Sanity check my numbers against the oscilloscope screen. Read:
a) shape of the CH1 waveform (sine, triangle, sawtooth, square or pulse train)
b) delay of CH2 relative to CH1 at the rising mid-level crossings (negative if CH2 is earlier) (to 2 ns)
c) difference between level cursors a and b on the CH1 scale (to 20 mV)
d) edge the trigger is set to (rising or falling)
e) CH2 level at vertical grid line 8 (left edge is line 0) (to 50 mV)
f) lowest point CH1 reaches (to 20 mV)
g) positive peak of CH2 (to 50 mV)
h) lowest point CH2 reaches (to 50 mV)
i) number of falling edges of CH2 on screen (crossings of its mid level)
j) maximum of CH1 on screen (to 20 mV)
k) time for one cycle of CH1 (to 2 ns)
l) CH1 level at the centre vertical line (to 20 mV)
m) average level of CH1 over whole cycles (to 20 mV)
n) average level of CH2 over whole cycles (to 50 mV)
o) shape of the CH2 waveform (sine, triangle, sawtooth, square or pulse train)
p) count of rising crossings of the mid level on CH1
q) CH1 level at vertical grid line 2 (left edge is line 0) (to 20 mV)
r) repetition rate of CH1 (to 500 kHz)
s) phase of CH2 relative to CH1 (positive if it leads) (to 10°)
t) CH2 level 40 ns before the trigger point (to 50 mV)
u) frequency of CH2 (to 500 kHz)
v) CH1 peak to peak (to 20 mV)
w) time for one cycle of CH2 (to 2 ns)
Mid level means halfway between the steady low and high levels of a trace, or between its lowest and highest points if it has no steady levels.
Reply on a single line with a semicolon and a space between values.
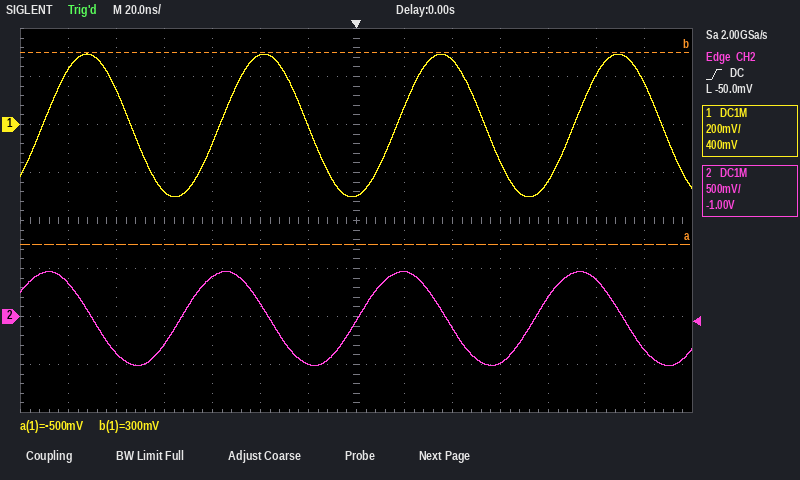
sine; -16 ns; 800 mV; rising; 450 mV; -300 mV; 450 mV; -500 mV; 4; 300 mV; 74 ns; -300 mV; 0 mV; 0 mV; sine; 4; 140 mV; 13.5 MHz; +80°; 150 mV; 13.5 MHz; 600 mV; 74 ns
